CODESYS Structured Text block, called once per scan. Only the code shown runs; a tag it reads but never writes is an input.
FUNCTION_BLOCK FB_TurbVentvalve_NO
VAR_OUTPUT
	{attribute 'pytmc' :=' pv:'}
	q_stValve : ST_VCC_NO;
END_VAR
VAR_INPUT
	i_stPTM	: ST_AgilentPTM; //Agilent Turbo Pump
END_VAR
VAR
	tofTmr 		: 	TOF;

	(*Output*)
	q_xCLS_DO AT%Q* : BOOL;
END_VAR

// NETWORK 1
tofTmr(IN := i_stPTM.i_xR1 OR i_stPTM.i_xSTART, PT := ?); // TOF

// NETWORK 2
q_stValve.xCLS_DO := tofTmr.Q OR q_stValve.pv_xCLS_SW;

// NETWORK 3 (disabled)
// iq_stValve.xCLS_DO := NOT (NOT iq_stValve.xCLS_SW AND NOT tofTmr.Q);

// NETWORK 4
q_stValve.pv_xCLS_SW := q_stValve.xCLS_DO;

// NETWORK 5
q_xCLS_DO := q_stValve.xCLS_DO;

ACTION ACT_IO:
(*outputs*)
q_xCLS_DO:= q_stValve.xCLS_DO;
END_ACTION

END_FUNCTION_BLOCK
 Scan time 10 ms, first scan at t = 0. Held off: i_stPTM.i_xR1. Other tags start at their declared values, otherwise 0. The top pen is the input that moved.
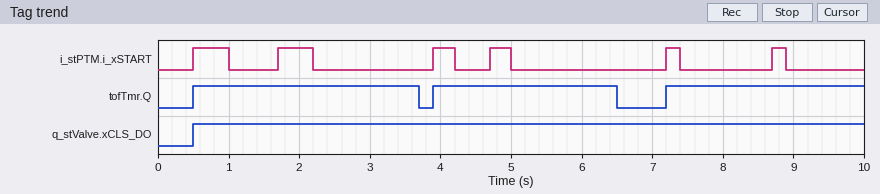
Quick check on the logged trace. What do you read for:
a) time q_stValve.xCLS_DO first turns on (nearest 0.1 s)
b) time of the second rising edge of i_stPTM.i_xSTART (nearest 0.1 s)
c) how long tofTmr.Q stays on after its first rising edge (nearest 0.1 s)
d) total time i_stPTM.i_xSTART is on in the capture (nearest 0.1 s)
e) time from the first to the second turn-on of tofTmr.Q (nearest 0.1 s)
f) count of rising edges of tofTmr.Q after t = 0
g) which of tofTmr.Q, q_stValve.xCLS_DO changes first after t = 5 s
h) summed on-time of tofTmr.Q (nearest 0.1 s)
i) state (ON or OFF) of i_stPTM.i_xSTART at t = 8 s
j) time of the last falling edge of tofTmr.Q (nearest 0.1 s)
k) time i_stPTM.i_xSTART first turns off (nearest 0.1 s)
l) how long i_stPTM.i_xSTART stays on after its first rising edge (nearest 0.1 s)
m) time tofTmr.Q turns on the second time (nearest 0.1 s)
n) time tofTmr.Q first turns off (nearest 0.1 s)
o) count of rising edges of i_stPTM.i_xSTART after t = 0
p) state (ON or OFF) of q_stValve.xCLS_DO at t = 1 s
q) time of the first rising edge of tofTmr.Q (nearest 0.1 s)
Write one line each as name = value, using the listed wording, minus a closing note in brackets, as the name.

time q_stValve.xCLS_DO first turns on = 0.5 s
time of the second rising edge of i_stPTM.i_xSTART = 1.7 s
how long tofTmr.Q stays on after its first rising edge = 3.2 s
total time i_stPTM.i_xSTART is on in the capture = 2.0 s
time from the first to the second turn-on of tofTmr.Q = 3.4 s
count of rising edges of tofTmr.Q after t = 0 = 3
which of tofTmr.Q, q_stValve.xCLS_DO changes first after t = 5 s = tofTmr.Q
summed on-time of tofTmr.Q = 8.6 s
state (ON or OFF) of i_stPTM.i_xSTART at t = 8 s = OFF
time of the last falling edge of tofTmr.Q = 6.5 s
time i_stPTM.i_xSTART first turns off = 1.0 s
how long i_stPTM.i_xSTART stays on after its first rising edge = 0.5 s
time tofTmr.Q turns on the second time = 3.9 s
time tofTmr.Q first turns off = 3.7 s
count of rising edges of i_stPTM.i_xSTART after t = 0 = 6
state (ON or OFF) of q_stValve.xCLS_DO at t = 1 s = ON
time of the first rising edge of tofTmr.Q = 0.5 s
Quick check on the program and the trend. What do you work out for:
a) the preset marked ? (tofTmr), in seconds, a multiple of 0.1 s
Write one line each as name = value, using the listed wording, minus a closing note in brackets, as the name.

the preset marked ? (tofTmr), in seconds, a multiple of 0.1 s = 1.5 s
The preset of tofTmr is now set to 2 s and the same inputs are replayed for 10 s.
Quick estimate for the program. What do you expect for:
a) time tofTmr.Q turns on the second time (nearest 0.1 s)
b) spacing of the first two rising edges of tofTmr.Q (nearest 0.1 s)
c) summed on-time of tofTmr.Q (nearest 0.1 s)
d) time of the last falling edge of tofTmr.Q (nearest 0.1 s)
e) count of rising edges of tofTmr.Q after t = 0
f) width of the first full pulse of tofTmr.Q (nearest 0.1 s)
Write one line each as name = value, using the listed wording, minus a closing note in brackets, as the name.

time tofTmr.Q turns on the second time = 7.2 s
spacing of the first two rising edges of tofTmr.Q = 6.7 s
summed on-time of tofTmr.Q = 9.3 s
time of the last falling edge of tofTmr.Q = 7.0 s
count of rising edges of tofTmr.Q after t = 0 = 2
width of the first full pulse of tofTmr.Q = 6.5 s
